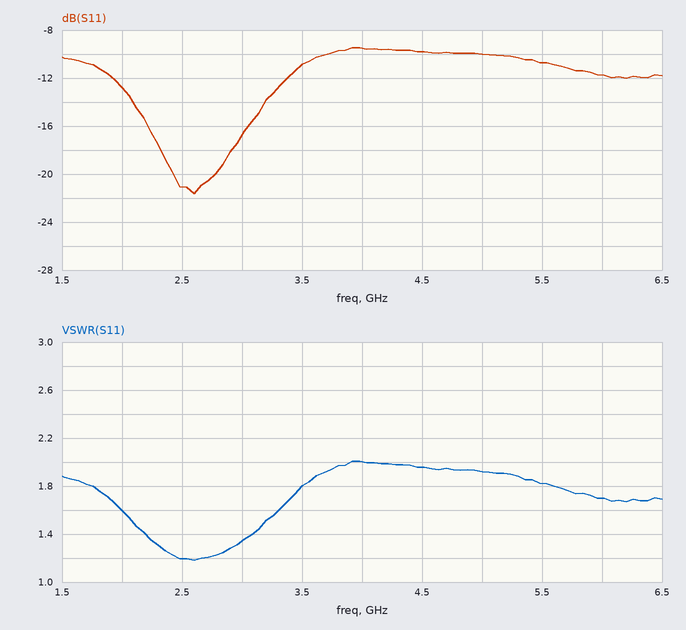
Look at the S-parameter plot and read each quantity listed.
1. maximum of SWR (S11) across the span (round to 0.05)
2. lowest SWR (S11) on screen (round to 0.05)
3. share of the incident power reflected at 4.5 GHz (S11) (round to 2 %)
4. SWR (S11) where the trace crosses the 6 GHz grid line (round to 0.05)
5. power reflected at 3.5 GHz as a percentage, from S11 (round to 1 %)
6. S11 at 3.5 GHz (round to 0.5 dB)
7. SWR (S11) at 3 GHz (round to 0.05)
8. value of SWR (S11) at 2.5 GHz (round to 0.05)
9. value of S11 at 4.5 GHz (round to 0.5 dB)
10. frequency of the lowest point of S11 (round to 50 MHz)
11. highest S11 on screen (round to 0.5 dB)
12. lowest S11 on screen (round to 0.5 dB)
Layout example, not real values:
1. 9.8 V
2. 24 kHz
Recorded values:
1. 2.00
2. 1.20
3. 10 %
4. 1.70
5. 8 %
6. -11.0 dB
7. 1.35
8. 1.20
9. -10.0 dB
10. 2.60 GHz
11. -9.5 dB
12. -21.5 dB
